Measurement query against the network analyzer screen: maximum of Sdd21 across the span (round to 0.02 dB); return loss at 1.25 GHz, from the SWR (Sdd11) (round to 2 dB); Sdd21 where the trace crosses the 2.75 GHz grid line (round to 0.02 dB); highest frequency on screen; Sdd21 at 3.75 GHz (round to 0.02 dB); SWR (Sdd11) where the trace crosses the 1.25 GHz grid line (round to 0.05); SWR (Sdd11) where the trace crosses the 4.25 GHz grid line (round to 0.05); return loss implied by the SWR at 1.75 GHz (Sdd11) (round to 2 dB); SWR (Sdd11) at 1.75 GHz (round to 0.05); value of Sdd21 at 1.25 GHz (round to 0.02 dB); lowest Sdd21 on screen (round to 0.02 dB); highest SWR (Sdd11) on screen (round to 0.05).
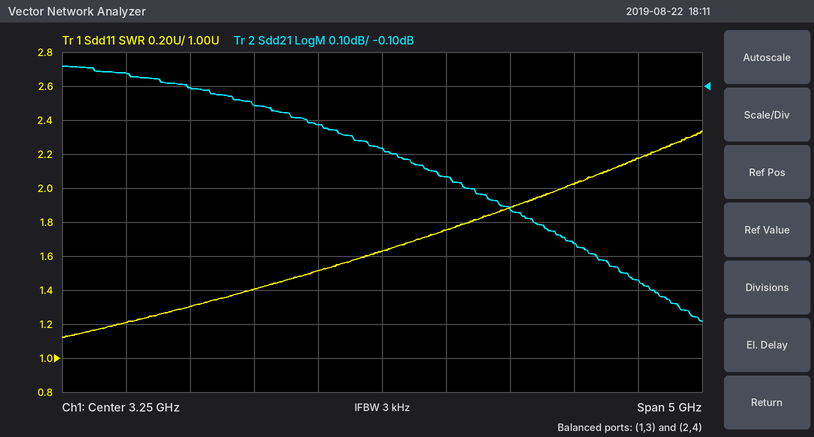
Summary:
-0.04 dB
20 dB
-0.22 dB
5.75 GHz
-0.36 dB
1.20
1.90
18 dB
1.30
-0.06 dB
-0.80 dB
2.35
